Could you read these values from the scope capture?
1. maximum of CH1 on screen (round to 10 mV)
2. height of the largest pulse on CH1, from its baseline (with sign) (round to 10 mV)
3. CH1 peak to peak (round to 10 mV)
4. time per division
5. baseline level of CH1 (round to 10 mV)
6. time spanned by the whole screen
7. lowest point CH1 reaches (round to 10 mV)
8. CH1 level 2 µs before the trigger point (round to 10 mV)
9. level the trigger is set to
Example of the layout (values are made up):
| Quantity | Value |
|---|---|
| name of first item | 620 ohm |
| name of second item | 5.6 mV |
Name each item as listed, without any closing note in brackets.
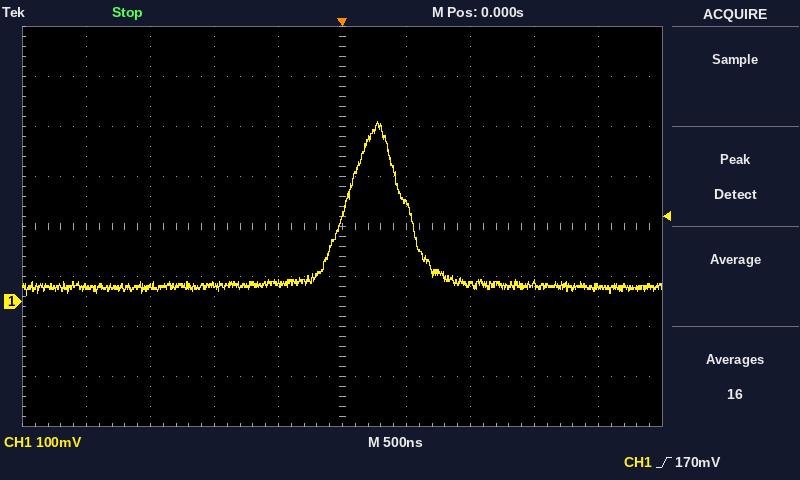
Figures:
| Quantity | Value |
|---|---|
| maximum of CH1 on screen | 360 mV |
| height of the largest pulse on CH1, from its baseline (with sign) | +330 mV |
| CH1 peak to peak | 350 mV |
| time per division | 500 ns |
| baseline level of CH1 | 30 mV |
| time spanned by the whole screen | 5 µs |
| lowest point CH1 reaches | 10 mV |
| CH1 level 2 µs before the trigger point | 30 mV |
| level the trigger is set to | 170 mV |
